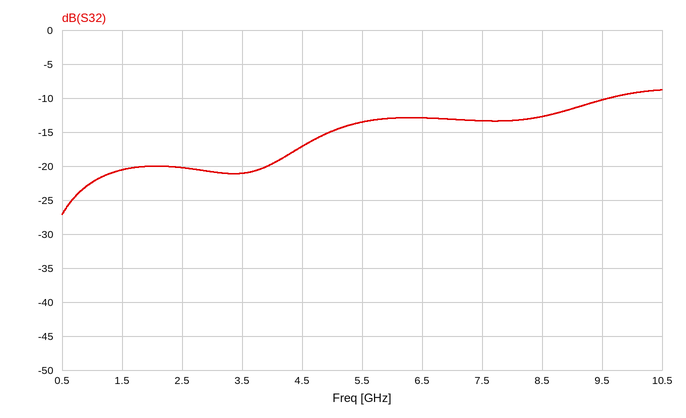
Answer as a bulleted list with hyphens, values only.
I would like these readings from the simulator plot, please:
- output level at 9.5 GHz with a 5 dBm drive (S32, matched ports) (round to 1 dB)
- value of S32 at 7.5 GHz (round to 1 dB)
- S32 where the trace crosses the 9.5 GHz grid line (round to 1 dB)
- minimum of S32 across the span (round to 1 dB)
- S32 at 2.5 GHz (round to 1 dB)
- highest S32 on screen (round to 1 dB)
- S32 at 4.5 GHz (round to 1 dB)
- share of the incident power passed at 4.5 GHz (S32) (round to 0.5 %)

- -5 dBm
- -13 dB
- -10 dB
- -27 dB
- -20 dB
- -9 dB
- -17 dB
- 2.0 %
